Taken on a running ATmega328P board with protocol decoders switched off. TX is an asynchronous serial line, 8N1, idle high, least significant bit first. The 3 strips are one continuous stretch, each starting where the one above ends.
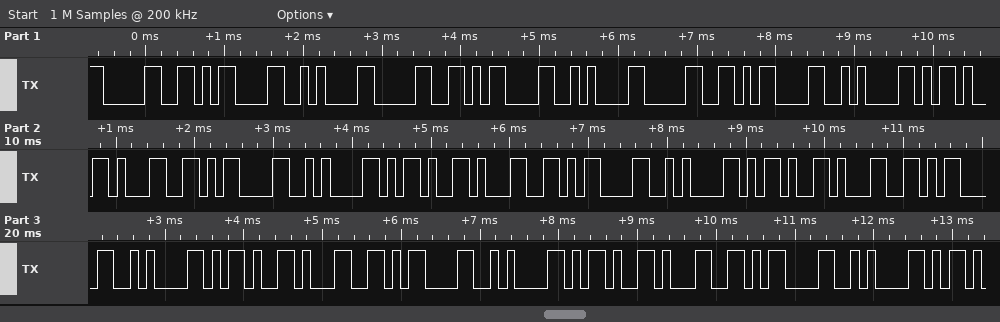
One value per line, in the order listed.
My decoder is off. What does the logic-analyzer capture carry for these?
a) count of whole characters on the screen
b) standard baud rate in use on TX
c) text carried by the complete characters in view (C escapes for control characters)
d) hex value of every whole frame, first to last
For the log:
29
9600 baud
"0\r\n0\r\n0\r\n-1\r\n-1\r\n-1\r\n-1\r\n-1\r\n"
30 0D 0A 30 0D 0A 30 0D 0A 2D 31 0D 0A 2D 31 0D 0A 2D 31 0D 0A 2D 31 0D 0A 2D 31 0D 0A
